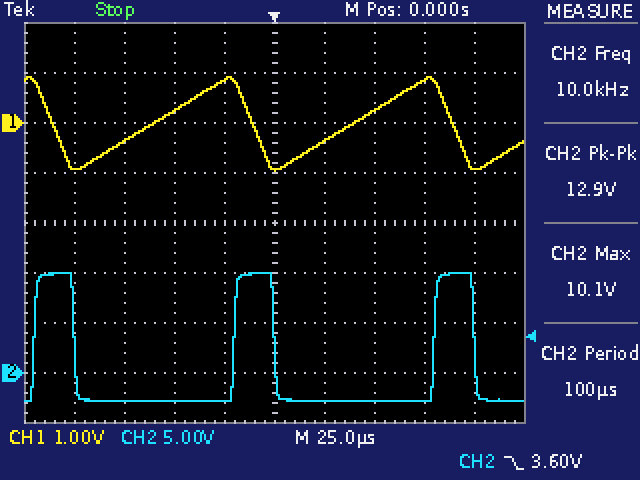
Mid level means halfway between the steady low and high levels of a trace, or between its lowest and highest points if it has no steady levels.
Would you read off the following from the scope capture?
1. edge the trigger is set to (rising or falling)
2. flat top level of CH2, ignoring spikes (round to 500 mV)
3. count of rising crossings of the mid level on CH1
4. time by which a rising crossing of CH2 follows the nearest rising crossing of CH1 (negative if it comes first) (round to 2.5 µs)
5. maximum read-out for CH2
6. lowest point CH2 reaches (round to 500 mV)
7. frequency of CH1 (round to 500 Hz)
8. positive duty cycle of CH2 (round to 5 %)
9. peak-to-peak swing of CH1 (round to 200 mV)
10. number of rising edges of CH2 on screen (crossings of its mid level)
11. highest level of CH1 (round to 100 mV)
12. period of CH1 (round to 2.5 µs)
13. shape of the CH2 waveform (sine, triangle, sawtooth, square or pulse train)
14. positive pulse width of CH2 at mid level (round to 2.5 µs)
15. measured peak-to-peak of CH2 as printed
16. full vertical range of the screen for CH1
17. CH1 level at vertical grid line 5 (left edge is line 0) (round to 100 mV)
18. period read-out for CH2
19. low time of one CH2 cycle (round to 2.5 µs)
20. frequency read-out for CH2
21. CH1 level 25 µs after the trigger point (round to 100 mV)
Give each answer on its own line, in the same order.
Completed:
falling
10.0 V
2
+40.0 µs
10.1 V
-3.0 V
10.0 kHz
20 %
1.8 V
3
900 mV
100.0 µs
pulse train
20.0 µs
12.9 V
8 V
-900 mV
100 µs
80.0 µs
10.0 kHz
-400 mV
